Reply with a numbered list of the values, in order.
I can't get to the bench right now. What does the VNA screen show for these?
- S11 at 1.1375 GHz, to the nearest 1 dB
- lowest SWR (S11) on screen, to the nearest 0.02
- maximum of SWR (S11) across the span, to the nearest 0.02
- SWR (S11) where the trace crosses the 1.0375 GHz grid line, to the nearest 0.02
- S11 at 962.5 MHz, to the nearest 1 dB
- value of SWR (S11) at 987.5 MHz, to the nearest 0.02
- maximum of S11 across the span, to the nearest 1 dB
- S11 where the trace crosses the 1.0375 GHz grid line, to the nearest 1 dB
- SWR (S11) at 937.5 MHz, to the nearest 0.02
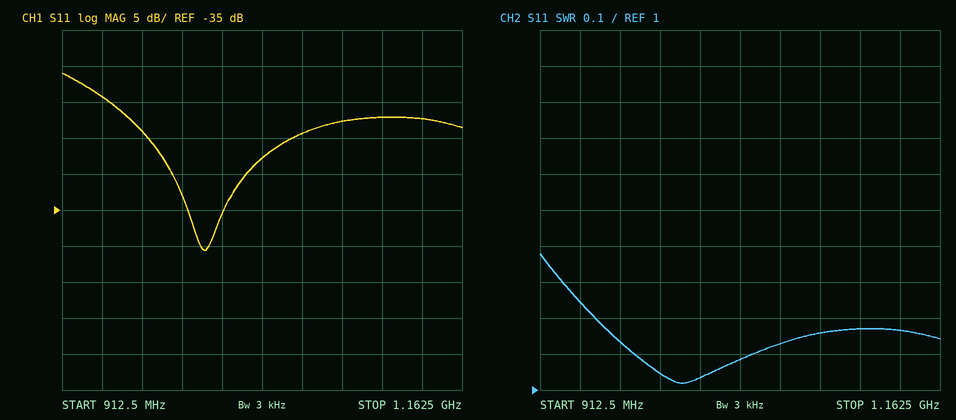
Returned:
1. -22 dB
2. 1.02
3. 1.38
4. 1.08
5. -24 dB
6. 1.04
7. -16 dB
8. -28 dB
9. 1.24
